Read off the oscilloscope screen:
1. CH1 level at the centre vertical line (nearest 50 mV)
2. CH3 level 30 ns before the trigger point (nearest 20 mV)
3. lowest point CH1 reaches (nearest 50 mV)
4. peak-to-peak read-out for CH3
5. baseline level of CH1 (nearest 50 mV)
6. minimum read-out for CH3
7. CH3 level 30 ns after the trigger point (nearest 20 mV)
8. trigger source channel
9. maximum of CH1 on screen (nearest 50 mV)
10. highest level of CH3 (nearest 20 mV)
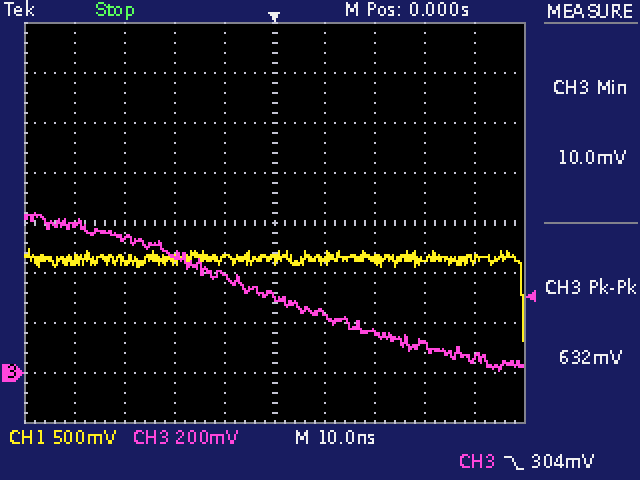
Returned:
1.15 V
540 mV
300 mV
632 mV
1.15 V
10.0 mV
120 mV
CH3
1.25 V
640 mV
